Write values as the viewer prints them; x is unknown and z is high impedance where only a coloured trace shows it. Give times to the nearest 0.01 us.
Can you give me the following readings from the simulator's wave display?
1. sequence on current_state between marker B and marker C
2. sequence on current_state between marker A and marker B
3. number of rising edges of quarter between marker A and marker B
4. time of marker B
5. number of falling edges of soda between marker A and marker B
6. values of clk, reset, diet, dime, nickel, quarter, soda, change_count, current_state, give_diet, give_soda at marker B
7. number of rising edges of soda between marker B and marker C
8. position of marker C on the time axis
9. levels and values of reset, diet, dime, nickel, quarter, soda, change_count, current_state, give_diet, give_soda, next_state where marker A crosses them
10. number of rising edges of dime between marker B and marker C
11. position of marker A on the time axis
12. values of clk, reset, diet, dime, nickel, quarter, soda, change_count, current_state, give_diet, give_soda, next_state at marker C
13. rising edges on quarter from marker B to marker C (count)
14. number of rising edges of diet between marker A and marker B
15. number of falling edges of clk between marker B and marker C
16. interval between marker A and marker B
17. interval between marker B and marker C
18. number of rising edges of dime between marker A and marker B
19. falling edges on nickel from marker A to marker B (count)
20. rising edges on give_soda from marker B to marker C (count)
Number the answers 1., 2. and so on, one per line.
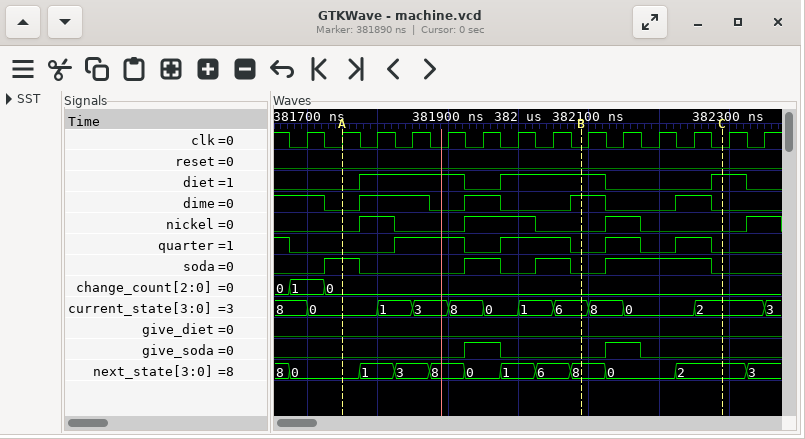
1. 6, 8, 0, 2
2. 0, 1, 3, 8, 0, 1, 6
3. 2
4. 382.09 us
5. 3
6. clk=0, reset=0, diet=1, dime=1, nickel=0, quarter=0, soda=0, change_count=0, current_state=6, give_diet=0, give_soda=0
7. 1
8. 382.29 us
9. reset=0, diet=0, dime=0, nickel=0, quarter=0, soda=1, change_count=0, current_state=0, give_diet=0, give_soda=0, next_state=0
10. 1
11. 381.75 us
12. clk=0, reset=0, diet=1, dime=0, nickel=0, quarter=0, soda=0, change_count=0, current_state=2, give_diet=0, give_soda=0, next_state=2
13. 2
14. 2
15. 4
16. 0.34 us
17. 0.2 us
18. 3
19. 2
20. 1
